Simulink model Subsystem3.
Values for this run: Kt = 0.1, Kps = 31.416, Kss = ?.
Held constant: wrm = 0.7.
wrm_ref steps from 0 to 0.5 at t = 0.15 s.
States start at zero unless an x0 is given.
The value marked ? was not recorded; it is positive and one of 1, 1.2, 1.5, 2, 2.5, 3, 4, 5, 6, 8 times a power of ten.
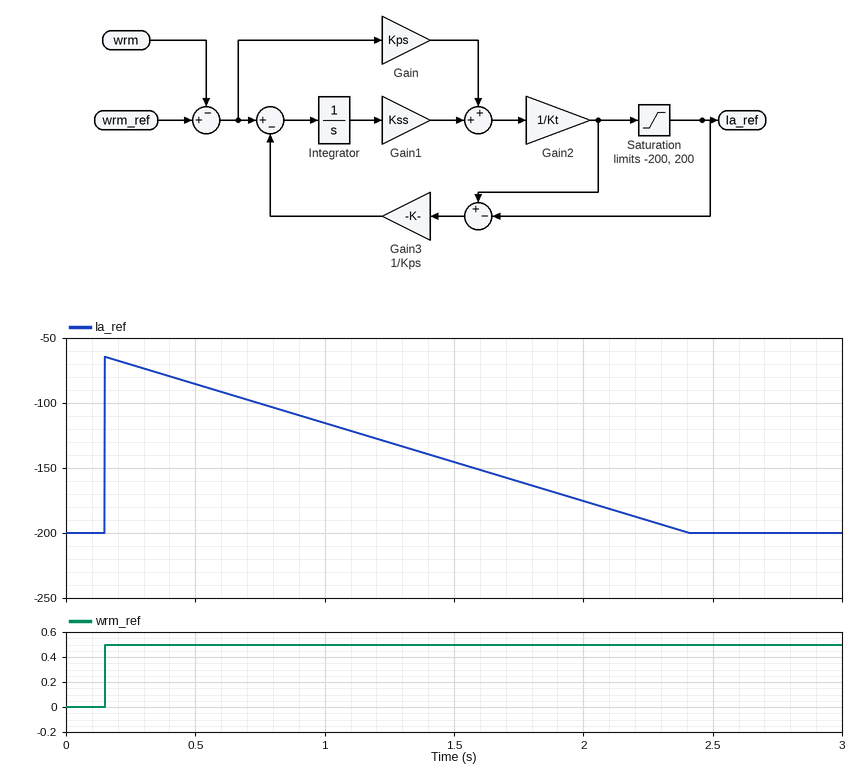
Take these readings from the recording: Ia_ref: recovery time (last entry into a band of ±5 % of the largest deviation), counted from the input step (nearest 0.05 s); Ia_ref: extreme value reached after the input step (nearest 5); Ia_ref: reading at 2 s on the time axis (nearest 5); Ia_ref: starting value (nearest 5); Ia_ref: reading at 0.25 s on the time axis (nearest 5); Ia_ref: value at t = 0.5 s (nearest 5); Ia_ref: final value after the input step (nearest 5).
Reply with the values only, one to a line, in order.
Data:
2.15 s
-65
-175
-200
-70
-85
-200
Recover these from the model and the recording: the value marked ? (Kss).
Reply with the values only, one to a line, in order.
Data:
30
